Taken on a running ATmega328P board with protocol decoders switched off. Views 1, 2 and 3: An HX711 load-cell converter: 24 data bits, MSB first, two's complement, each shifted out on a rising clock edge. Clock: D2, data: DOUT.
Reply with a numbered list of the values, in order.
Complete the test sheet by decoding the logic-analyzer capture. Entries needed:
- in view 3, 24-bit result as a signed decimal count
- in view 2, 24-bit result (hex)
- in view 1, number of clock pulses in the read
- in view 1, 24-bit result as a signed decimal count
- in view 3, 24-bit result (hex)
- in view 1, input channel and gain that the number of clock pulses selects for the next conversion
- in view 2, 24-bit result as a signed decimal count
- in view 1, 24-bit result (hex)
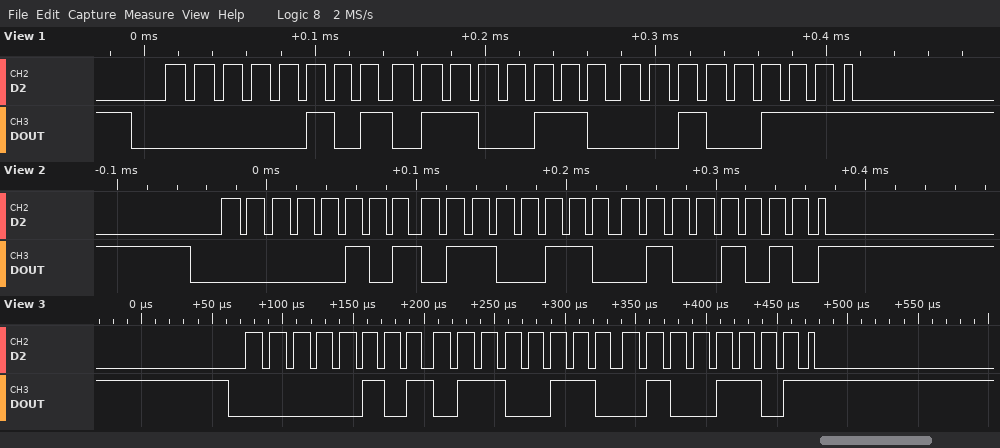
1. 353869
2. 0x05664A
3. 25
4. 353831
5. 0x05664D
6. channel A, gain 128
7. 353866
8. 0x056627
